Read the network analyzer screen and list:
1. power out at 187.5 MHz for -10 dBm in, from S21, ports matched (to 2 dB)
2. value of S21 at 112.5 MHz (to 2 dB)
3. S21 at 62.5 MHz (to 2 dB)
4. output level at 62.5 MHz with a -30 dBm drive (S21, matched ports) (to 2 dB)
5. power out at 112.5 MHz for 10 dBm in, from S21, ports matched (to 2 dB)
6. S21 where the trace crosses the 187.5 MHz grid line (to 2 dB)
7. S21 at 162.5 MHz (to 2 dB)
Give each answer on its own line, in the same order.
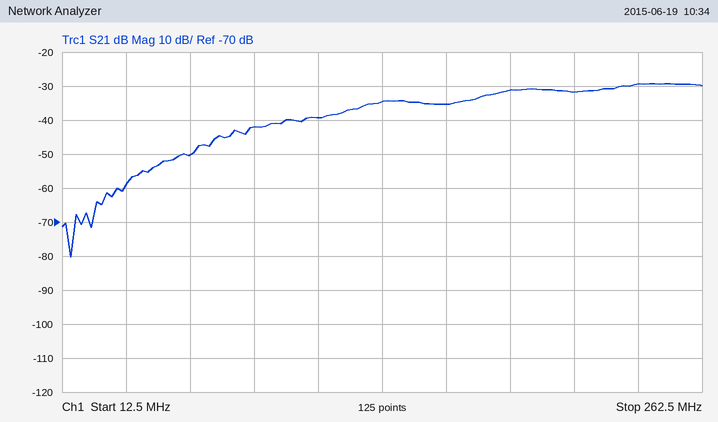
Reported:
-42 dBm
-40 dB
-50 dB
-80 dBm
-30 dBm
-32 dB
-36 dB
